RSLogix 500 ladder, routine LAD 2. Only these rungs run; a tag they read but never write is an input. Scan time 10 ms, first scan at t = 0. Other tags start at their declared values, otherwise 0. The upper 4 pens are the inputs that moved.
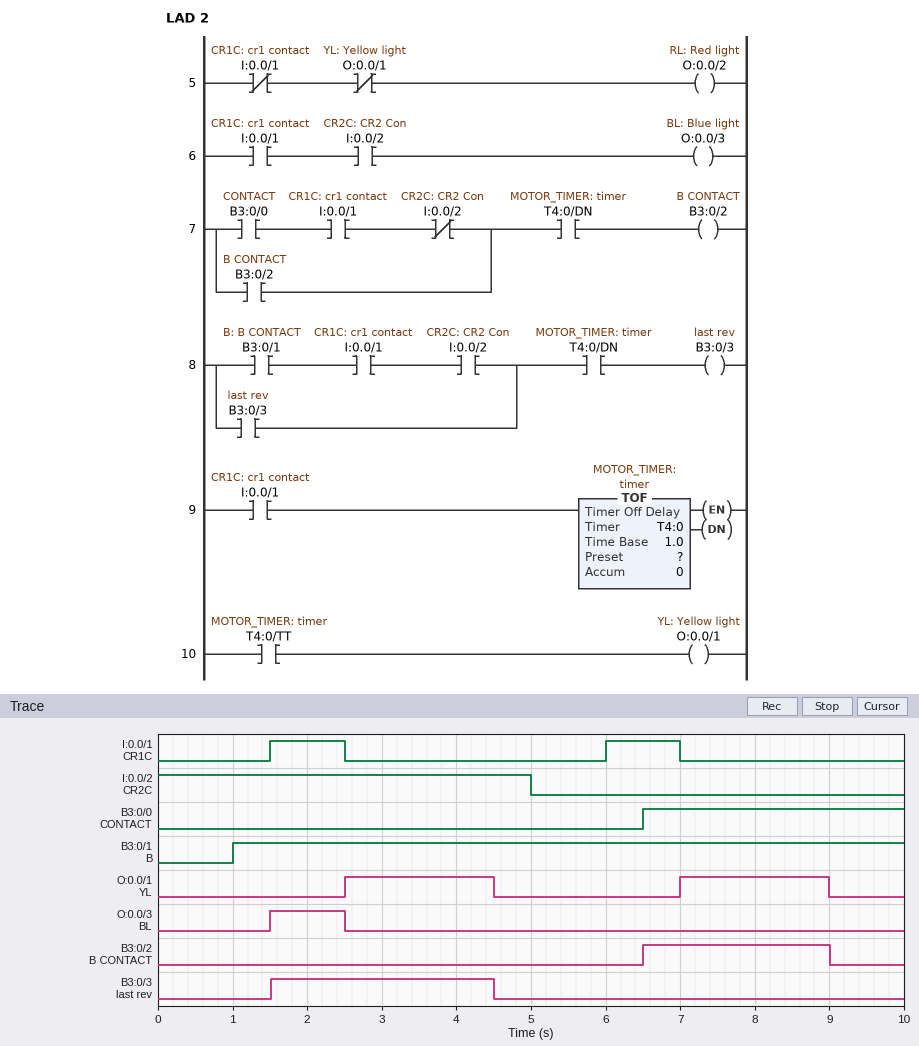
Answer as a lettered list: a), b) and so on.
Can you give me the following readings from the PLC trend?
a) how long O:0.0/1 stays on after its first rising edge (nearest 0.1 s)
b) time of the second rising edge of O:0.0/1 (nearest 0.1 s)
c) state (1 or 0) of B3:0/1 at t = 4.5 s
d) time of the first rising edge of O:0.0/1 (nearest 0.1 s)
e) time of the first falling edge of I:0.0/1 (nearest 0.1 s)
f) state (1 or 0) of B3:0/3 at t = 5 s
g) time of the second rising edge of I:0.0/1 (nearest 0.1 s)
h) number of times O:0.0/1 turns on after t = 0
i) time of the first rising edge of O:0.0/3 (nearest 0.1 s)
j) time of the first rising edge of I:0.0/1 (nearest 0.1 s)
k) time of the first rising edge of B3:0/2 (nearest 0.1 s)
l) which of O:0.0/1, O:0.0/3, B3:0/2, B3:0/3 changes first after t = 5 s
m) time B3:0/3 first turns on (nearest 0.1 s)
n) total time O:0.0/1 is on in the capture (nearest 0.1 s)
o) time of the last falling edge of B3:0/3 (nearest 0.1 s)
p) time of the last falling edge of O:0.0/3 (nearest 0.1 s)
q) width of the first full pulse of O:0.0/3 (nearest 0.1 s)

a) 2.0 s
b) 7.0 s
c) 1
d) 2.5 s
e) 2.5 s
f) 0
g) 6.0 s
h) 2
i) 1.5 s
j) 1.5 s
k) 6.5 s
l) B3:0/2
m) 1.5 s
n) 4.0 s
o) 4.5 s
p) 2.5 s
q) 1.0 s
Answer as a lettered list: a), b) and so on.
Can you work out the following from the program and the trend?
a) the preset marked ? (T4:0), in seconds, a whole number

a) 2 s
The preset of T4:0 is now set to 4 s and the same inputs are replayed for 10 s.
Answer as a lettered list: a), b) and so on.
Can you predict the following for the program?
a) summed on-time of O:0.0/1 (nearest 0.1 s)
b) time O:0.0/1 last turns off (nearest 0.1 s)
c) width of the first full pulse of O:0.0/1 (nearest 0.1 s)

a) 6.5 s
b) 6.0 s
c) 3.5 s
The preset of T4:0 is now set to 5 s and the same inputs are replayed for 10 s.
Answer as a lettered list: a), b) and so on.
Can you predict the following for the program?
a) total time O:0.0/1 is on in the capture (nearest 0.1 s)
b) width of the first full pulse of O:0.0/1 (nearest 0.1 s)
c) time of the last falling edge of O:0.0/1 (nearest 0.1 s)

a) 6.5 s
b) 3.5 s
c) 6.0 s
